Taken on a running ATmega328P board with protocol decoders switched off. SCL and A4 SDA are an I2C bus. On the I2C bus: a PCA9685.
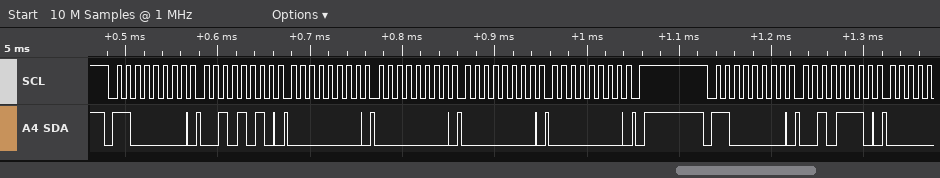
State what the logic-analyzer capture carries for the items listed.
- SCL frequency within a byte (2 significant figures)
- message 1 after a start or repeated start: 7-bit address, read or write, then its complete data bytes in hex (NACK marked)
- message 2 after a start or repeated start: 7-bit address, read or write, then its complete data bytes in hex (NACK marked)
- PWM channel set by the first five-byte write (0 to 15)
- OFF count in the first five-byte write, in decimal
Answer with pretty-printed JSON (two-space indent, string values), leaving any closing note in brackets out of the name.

{
  "SCL frequency within a byte": "100 kHz",
  "message 1 after a start or repeated start: 7-bit address, read or write, then its complete data bytes in hex": "0x60 write: 2A 00 00 00 00",
  "message 2 after a start or repeated start: 7-bit address, read or write, then its complete data bytes in hex": "0x60 write: 2E",
  "PWM channel set by the first five-byte write": "9",
  "OFF count in the first five-byte write, in decimal": "0"
}
